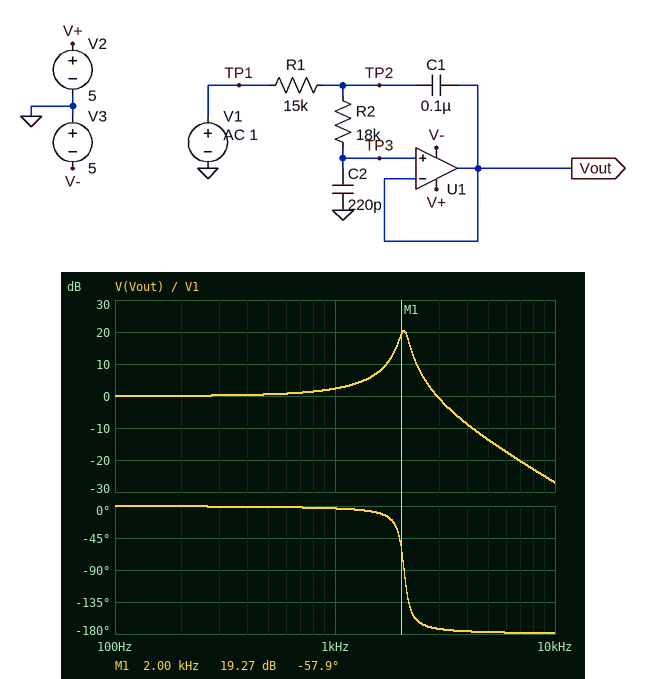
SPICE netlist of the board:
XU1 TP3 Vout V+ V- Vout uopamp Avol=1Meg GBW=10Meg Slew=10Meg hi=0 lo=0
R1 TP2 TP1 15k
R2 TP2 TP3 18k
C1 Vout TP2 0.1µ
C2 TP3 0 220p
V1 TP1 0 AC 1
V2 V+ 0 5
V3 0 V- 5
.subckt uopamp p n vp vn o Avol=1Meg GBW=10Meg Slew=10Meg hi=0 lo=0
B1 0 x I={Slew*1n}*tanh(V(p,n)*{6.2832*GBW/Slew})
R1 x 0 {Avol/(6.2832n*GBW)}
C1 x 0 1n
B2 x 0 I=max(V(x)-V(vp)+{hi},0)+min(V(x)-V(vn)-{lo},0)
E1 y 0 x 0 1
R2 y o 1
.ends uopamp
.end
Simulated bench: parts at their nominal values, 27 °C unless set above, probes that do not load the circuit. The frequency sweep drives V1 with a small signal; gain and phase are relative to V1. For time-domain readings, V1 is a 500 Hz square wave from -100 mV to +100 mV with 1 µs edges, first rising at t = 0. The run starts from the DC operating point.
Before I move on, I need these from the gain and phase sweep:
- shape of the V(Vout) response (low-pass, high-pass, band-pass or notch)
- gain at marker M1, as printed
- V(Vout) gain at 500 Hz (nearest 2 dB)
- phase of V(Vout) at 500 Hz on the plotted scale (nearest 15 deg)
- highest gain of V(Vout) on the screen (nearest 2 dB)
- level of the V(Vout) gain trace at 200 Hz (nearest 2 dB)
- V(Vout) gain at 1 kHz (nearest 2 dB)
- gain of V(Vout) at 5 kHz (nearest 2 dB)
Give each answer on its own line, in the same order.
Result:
low-pass
19.27 dB
0 dB
0 deg
20 dB
0 dB
2 dB
-14 dB
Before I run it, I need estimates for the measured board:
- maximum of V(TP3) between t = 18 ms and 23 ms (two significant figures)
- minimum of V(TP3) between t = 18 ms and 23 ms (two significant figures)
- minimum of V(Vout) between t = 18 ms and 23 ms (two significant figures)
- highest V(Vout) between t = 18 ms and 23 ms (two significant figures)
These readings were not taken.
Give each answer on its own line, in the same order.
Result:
210 mV
-210 mV
-210 mV
210 mV
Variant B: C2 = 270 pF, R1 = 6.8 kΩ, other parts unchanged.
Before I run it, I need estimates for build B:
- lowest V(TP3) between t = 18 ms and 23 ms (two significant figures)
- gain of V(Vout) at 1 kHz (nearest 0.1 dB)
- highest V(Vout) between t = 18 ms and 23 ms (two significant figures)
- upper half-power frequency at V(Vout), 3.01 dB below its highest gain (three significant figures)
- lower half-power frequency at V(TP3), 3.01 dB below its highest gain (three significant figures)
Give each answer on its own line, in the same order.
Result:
-260 mV
1.2 dB
260 mV
2.91 kHz
2.59 kHz
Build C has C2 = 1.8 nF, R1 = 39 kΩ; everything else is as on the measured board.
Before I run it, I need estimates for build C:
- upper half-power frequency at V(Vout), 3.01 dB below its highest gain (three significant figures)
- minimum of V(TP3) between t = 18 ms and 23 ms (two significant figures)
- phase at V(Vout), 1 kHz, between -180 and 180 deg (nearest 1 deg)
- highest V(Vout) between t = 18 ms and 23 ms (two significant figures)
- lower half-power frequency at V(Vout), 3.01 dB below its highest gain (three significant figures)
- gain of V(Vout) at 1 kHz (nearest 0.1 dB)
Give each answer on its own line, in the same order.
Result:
499 Hz
-320 mV
-171 deg
320 mV
367 Hz
-12.1 dB
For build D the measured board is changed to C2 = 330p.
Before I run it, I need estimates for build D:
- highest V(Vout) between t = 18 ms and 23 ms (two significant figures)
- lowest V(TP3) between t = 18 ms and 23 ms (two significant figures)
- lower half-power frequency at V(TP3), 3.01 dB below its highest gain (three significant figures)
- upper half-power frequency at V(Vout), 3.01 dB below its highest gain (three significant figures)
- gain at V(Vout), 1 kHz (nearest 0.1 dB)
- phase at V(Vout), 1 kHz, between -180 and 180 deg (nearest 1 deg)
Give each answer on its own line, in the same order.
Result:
290 mV
-290 mV
1.58 kHz
1.77 kHz
3.7 dB
-6 deg
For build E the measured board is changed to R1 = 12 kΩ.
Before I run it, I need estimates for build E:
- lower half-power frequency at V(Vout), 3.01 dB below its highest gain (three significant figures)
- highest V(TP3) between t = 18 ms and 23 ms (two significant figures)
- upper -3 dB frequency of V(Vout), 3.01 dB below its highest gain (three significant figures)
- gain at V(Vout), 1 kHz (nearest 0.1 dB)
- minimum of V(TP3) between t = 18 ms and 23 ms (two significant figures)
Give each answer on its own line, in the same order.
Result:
2.19 kHz
270 mV
2.41 kHz
1.8 dB
-270 mV
